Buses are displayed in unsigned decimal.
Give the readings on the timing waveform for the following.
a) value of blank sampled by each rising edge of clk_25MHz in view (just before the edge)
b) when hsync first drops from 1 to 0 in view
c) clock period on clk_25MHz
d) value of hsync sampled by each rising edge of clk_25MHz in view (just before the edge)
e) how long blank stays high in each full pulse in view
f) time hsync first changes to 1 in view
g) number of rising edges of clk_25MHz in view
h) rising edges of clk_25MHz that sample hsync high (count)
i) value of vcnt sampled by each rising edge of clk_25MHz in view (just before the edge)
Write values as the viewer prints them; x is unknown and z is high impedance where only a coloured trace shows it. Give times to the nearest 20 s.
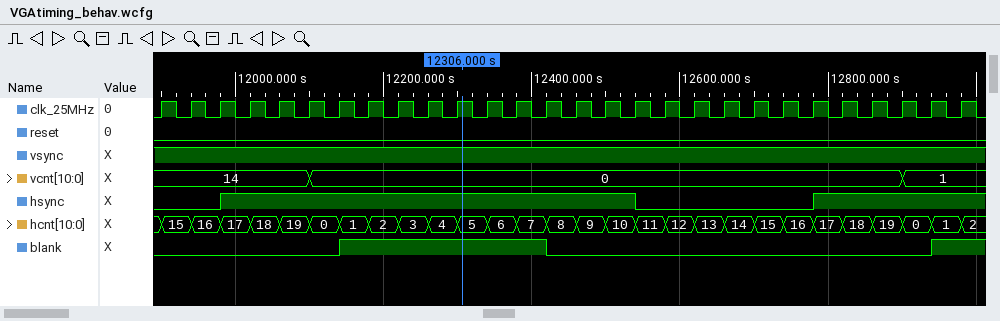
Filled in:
0 0 0 0 0 0 0 1 1 1 1 1 1 1 0 0 0 0 0 0 0 0 0 0 0 0 0 1
12540 s
40 s
0 0 0 1 1 1 1 1 1 1 1 1 1 1 1 1 1 0 0 0 0 0 0 1 1 1 1 1
280 s
11980 s
28
19
14, 14, 14, 14, 14, 14, 0, 0, 0, 0, 0, 0, 0, 0, 0, 0, 0, 0, 0, 0, 0, 0, 0, 0, 0, 0, 1, 1
